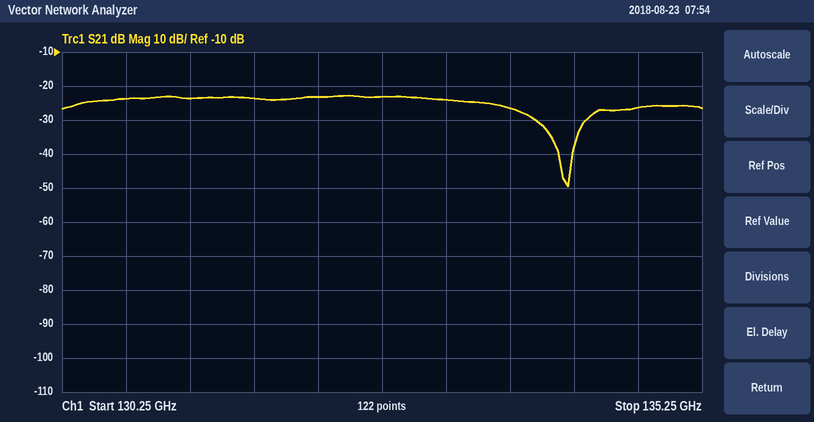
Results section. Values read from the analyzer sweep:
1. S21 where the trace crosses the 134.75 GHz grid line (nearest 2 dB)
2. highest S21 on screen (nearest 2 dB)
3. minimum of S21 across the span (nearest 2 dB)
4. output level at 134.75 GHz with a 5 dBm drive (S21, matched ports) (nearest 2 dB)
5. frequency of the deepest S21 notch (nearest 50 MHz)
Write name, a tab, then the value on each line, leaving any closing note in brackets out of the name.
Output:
S21 where the trace crosses the 134.75 GHz grid line	-26 dB
highest S21 on screen	-22 dB
minimum of S21 across the span	-50 dB
output level at 134.75 GHz with a 5 dBm drive (S21, matched ports)	-22 dBm
frequency of the deepest S21 notch	134.20 GHz
